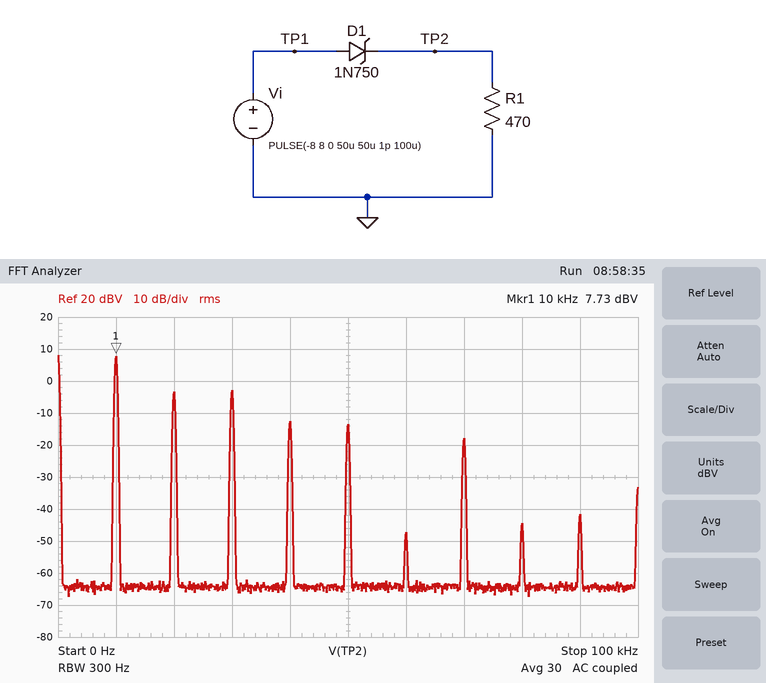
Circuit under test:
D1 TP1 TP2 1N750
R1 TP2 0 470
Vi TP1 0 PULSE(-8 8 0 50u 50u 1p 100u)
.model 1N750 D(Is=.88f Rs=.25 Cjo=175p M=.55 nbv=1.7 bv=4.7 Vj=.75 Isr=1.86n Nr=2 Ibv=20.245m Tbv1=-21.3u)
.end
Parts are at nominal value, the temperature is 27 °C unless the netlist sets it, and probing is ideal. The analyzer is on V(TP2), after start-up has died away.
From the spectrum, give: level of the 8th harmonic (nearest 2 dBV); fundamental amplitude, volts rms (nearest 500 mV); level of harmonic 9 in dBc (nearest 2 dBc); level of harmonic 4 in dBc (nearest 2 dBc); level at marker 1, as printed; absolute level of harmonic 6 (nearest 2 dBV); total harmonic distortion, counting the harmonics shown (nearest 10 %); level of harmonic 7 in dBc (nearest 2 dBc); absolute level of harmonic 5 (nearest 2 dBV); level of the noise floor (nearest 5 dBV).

-44 dBV
2.5 V
-50 dBc
-20 dBc
7.73 dBV
-48 dBV
40 %
-26 dBc
-14 dBV
-65 dBV
